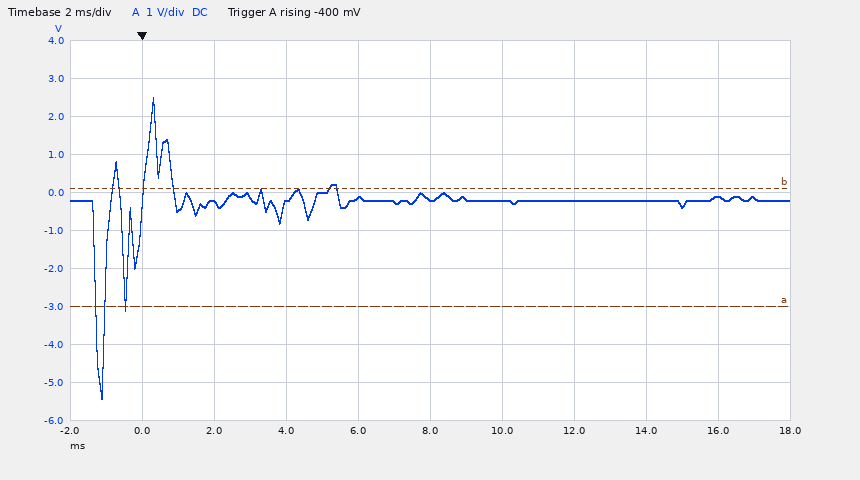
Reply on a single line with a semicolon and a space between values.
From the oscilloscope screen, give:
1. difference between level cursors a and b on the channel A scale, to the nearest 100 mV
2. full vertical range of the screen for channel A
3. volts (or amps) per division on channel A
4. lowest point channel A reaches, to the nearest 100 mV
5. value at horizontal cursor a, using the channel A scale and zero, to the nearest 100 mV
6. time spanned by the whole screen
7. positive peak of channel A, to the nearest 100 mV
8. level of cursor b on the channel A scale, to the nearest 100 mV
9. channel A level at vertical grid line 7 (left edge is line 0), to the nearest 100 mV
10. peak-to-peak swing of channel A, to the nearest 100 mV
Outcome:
3.1 V; 10 V; 1 V; -5.4 V; -3.0 V; 20 ms; 2.5 V; 100 mV; -200 mV; 7.9 V
